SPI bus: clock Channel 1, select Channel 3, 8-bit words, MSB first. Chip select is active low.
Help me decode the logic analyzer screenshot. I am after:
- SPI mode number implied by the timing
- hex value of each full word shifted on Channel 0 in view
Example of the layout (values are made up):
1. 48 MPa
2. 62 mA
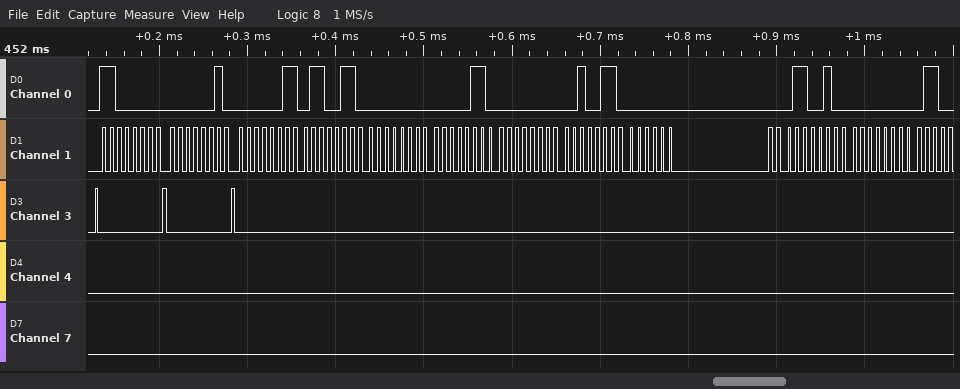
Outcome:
1. 0
2. C0, 02, 03, 66, 00, 06, 00, 26, 00, 64, 00
